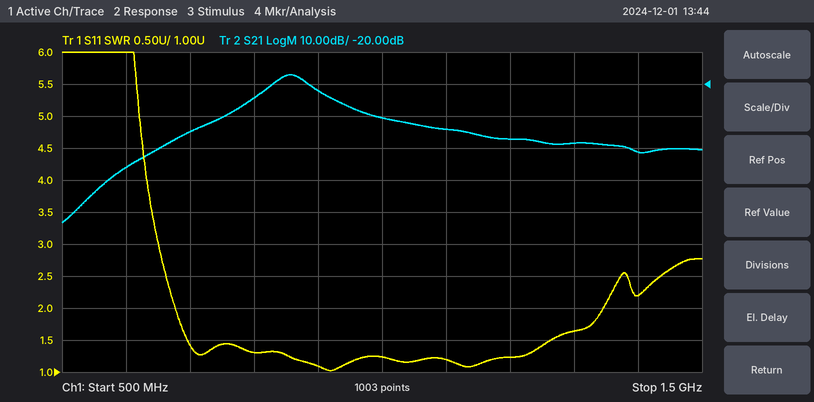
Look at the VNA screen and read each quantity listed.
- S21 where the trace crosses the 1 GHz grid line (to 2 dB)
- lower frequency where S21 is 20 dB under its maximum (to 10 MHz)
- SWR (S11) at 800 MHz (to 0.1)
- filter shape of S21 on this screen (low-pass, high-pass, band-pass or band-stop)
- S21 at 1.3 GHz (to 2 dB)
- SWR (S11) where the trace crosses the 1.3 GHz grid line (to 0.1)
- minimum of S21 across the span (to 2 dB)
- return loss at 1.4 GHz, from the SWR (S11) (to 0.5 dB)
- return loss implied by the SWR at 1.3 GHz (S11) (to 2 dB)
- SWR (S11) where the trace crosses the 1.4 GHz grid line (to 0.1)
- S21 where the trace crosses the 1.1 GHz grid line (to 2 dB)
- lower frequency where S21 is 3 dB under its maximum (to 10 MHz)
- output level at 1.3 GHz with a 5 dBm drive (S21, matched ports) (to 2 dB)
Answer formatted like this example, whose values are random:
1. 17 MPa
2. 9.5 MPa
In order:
1. -30 dB
2. 680 MHz
3. 1.3
4. band-pass
5. -38 dB
6. 1.6
7. -64 dB
8. 8.5 dB
9. 12 dB
10. 2.2
11. -34 dB
12. 830 MHz
13. -34 dBm
